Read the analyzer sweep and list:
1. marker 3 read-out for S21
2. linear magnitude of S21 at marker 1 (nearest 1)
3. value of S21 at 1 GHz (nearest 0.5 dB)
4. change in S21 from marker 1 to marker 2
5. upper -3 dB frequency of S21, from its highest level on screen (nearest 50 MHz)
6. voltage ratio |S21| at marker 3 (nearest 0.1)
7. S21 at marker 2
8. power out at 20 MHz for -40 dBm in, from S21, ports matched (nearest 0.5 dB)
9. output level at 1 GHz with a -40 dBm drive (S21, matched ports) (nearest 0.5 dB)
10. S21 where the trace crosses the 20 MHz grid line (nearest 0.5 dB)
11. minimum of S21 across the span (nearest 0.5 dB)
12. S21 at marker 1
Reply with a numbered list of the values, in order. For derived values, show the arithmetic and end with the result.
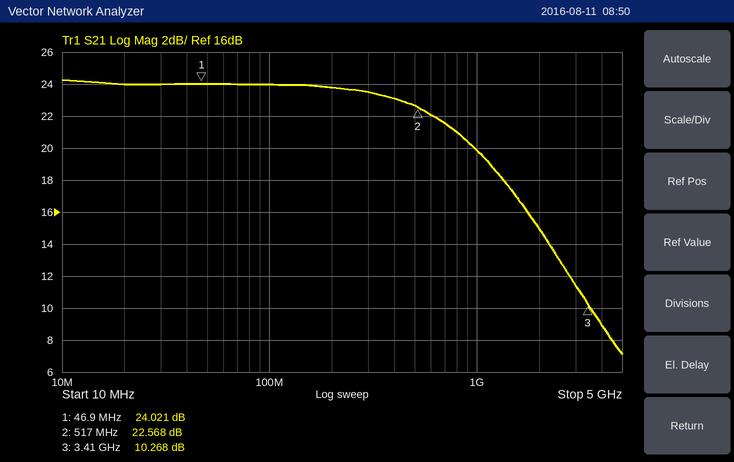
1. 10.268 dB
2. 10^(24.021/20) ≈ 16
3. 20.0 dB
4. 22.568 − (24.021) = -1.453 dB
5. 750 MHz
6. 10^(10.268/20) ≈ 3.3
7. 22.568 dB
8. -40 dBm + (24.0 dB) = -16.0 dBm
9. -40 dBm + (20.0 dB) = -20.0 dBm
10. 24.0 dB
11. 7.0 dB
12. 24.021 dB
